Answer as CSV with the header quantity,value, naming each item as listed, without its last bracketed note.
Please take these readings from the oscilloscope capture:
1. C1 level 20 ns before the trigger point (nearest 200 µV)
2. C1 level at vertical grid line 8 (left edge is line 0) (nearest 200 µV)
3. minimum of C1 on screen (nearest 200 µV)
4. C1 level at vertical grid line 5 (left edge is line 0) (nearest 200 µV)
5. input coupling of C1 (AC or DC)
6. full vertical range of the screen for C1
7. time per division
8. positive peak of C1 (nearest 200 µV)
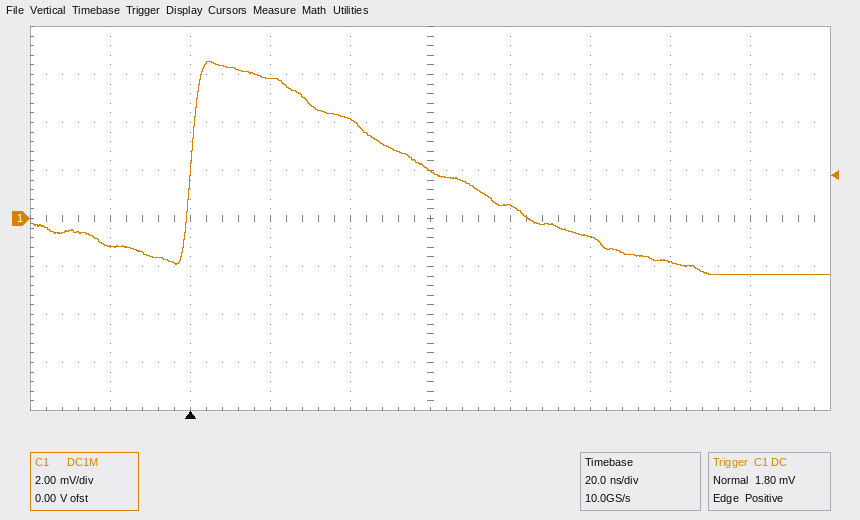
quantity,value
C1 level 20 ns before the trigger point,-1.2 mV
C1 level at vertical grid line 8 (left edge is line 0),-1.8 mV
minimum of C1 on screen,-2.4 mV
C1 level at vertical grid line 5 (left edge is line 0),2.0 mV
input coupling of C1,DC
full vertical range of the screen for C1,16 mV
time per division,20 ns
positive peak of C1,6.6 mV
